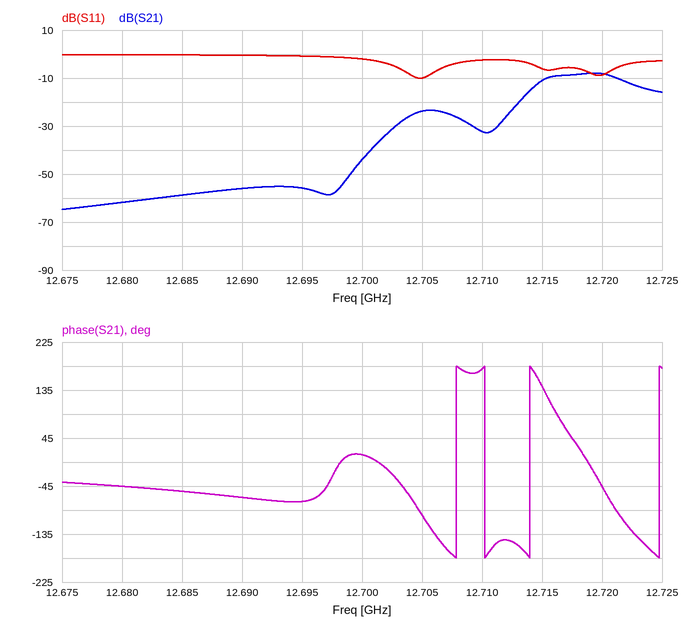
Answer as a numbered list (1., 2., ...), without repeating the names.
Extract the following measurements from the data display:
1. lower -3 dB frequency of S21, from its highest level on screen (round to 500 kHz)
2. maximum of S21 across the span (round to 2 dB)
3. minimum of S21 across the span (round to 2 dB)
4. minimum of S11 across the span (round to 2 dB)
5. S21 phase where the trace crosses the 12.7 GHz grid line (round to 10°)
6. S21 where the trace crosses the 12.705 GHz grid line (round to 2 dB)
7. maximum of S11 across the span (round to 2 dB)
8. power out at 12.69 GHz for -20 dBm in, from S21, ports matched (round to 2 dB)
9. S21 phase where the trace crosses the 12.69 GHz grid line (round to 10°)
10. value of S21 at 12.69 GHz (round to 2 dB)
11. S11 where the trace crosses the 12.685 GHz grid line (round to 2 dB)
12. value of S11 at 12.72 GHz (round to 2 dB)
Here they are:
1. 12.7150 GHz
2. -8 dB
3. -64 dB
4. -10 dB
5. 10°
6. -24 dB
7. 0 dB
8. -76 dBm
9. -70°
10. -56 dB
11. 0 dB
12. -8 dB
